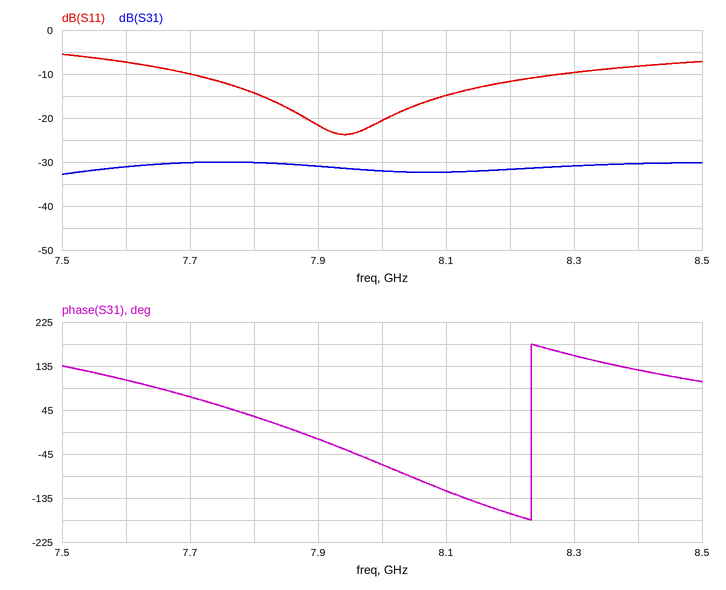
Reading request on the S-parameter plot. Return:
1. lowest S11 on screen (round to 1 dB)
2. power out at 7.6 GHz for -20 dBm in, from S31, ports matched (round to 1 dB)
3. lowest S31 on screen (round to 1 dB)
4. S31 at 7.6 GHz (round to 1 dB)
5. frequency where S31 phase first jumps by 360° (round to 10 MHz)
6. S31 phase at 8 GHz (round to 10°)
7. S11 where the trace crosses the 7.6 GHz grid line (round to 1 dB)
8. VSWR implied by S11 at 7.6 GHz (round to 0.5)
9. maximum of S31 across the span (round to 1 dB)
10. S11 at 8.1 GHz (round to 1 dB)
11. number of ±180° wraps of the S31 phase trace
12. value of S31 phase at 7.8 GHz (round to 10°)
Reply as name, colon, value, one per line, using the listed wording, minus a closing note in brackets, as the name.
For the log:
lowest S11 on screen: -24 dB
power out at 7.6 GHz for -20 dBm in, from S31, ports matched: -51 dBm
lowest S31 on screen: -33 dB
S31 at 7.6 GHz: -31 dB
frequency where S31 phase first jumps by 360°: 8.23 GHz
S31 phase at 8 GHz: -70°
S11 where the trace crosses the 7.6 GHz grid line: -7 dB
VSWR implied by S11 at 7.6 GHz: 2.5
maximum of S31 across the span: -30 dB
S11 at 8.1 GHz: -15 dB
number of ±180° wraps of the S31 phase trace: 1
value of S31 phase at 7.8 GHz: 30°
